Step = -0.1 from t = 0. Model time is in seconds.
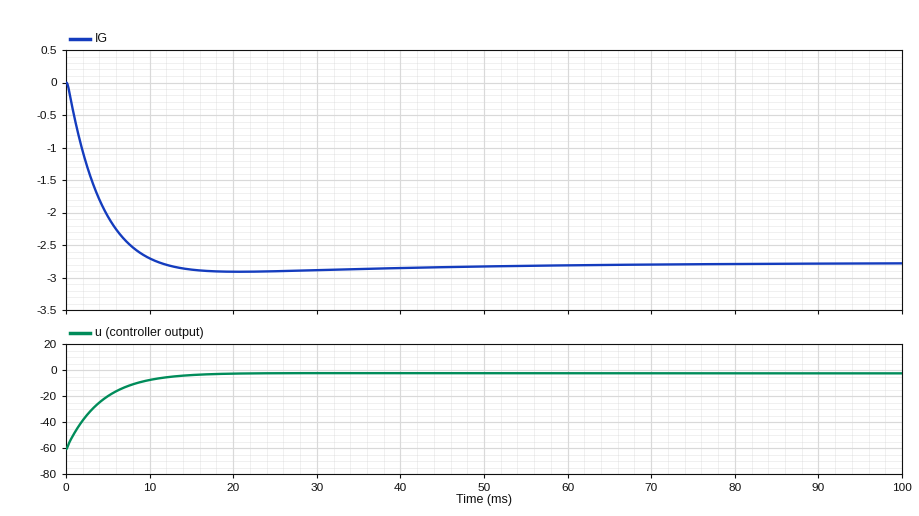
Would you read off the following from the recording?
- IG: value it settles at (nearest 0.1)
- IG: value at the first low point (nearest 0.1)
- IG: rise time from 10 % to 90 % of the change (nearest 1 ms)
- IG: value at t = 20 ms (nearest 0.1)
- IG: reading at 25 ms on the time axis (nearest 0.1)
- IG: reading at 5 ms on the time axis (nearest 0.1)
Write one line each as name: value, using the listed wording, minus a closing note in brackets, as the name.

IG: value it settles at: -2.8
IG: value at the first low point: -2.9
IG: rise time from 10 % to 90 % of the change: 7 ms
IG: value at t = 20 ms: -2.9
IG: reading at 25 ms on the time axis: -2.9
IG: reading at 5 ms on the time axis: -2.1
